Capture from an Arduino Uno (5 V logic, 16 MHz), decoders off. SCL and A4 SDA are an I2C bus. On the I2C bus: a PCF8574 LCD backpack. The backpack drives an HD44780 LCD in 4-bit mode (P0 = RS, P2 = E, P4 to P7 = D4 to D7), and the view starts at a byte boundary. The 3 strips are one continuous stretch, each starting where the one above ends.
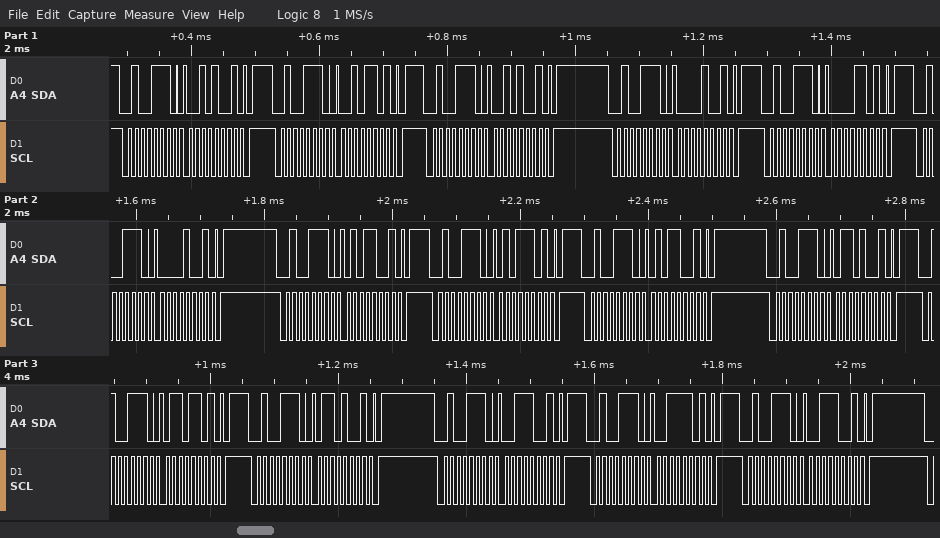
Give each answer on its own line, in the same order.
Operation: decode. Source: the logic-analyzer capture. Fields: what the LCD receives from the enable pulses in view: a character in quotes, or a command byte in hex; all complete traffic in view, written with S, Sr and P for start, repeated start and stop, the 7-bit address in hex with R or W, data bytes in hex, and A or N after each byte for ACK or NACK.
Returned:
' ' 'V'
S 27W A 29 A P S 27W A 2D A P S 27W A 29 A P S 27W A 09 A P S 27W A 0D A P S 27W A 09 A P S 27W A 59 A P S 27W A 5D A P S 27W A 59 A P S 27W A 69 A P S 27W A 6D A P S 27W A 69 A P S 27W A 39 A P S 27W A 3D A P S 27W A 39 A P
